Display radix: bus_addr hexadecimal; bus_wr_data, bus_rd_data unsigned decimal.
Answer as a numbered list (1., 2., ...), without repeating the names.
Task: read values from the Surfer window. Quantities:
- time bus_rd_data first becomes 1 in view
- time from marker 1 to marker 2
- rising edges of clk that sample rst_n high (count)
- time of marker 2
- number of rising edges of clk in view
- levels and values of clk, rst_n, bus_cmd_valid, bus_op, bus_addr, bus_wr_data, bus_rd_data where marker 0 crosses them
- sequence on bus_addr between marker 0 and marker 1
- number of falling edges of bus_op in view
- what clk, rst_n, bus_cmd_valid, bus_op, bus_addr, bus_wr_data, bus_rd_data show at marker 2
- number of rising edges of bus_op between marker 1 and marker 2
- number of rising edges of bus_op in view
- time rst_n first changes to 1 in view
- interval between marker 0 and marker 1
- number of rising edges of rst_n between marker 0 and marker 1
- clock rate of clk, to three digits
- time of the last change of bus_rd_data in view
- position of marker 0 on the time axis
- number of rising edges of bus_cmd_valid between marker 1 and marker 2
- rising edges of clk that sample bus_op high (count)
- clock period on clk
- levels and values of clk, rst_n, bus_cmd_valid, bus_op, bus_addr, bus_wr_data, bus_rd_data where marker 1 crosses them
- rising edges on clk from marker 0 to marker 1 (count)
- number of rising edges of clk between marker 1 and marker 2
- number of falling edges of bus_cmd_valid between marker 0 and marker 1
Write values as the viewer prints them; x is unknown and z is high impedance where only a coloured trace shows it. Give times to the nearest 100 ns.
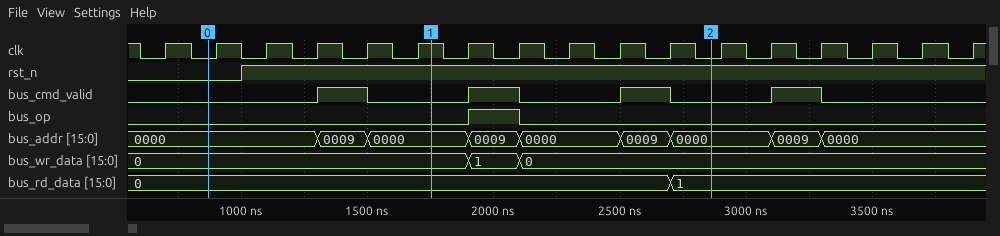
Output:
1. 2700 ns
2. 1100 ns
3. 15
4. 2900 ns
5. 17
6. clk=0, rst_n=0, bus_cmd_valid=0, bus_op=0, bus_addr=0000, bus_wr_data=0, bus_rd_data=0
7. 0000, 0009, 0000
8. 1
9. clk=0, rst_n=1, bus_cmd_valid=0, bus_op=0, bus_addr=0000, bus_wr_data=0, bus_rd_data=1
10. 1
11. 1
12. 1000 ns
13. 900 ns
14. 1
15. 5.00 MHz
16. 2700 ns
17. 900 ns
18. 2
19. 1
20. 200 ns
21. clk=1, rst_n=1, bus_cmd_valid=0, bus_op=0, bus_addr=0000, bus_wr_data=0, bus_rd_data=0
22. 5
23. 5
24. 1
